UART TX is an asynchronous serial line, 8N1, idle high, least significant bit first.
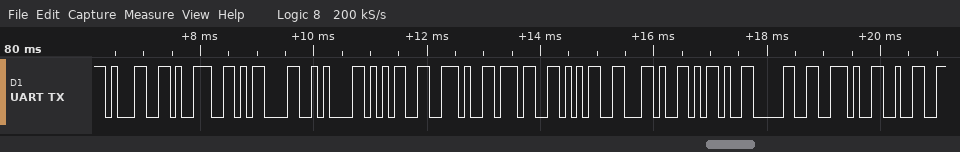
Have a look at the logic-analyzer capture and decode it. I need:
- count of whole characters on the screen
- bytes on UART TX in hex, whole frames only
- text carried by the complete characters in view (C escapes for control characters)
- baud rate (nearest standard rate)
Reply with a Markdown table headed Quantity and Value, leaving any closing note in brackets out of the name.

| Quantity | Value |
|---|---|
| count of whole characters on the screen | 13 |
| bytes on UART TX in hex, whole frames only | 31 39 0D 0A 35 2E 37 35 2C 2D 30 2E 32 |
| text carried by the complete characters in view | "19\r\n5.75,-0.2" |
| baud rate | 9600 baud |
